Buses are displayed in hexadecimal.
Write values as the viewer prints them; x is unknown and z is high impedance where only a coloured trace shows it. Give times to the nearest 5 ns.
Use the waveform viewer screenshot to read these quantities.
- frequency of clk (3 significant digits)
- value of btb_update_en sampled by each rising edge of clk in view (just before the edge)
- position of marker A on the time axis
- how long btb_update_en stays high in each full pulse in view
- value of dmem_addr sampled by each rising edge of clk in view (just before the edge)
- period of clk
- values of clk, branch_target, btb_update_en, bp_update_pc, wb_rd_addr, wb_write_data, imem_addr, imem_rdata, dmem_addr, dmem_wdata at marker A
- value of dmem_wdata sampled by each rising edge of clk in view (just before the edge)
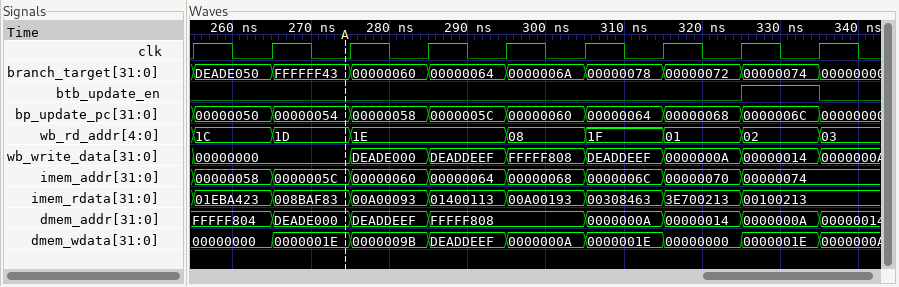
100 MHz
0 0 0 0 0 0 0 0 1
275 ns
10 ns
FFFFF804, FFFFF804, DEADE000, DEADDEEF, FFFFF808, FFFFF808, 0000000A, 00000014, 0000000A
10 ns
clk=0, branch_target=FFFFFF43, btb_update_en=0, bp_update_pc=00000054, wb_rd_addr=1D, wb_write_data=00000000, imem_addr=0000005C, imem_rdata=008BAF83, dmem_addr=DEADE000, dmem_wdata=0000001E
00000000, 00000000, 0000001E, 0000009B, DEADDEEF, 0000000A, 0000001E, 00000000, 0000001E
